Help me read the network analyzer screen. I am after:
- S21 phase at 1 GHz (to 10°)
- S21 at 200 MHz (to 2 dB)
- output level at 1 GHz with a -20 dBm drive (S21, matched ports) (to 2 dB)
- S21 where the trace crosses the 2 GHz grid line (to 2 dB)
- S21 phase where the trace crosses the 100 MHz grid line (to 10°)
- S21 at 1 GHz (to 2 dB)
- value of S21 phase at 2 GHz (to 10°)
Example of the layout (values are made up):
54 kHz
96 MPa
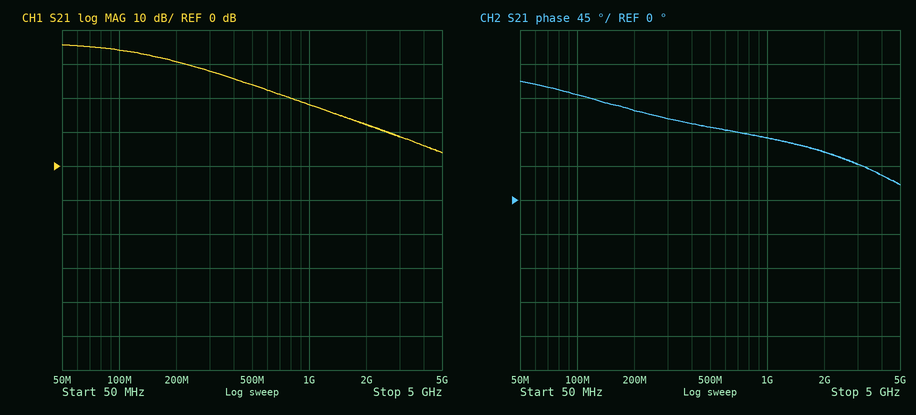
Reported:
80°
30 dB
-2 dBm
12 dB
140°
18 dB
60°
